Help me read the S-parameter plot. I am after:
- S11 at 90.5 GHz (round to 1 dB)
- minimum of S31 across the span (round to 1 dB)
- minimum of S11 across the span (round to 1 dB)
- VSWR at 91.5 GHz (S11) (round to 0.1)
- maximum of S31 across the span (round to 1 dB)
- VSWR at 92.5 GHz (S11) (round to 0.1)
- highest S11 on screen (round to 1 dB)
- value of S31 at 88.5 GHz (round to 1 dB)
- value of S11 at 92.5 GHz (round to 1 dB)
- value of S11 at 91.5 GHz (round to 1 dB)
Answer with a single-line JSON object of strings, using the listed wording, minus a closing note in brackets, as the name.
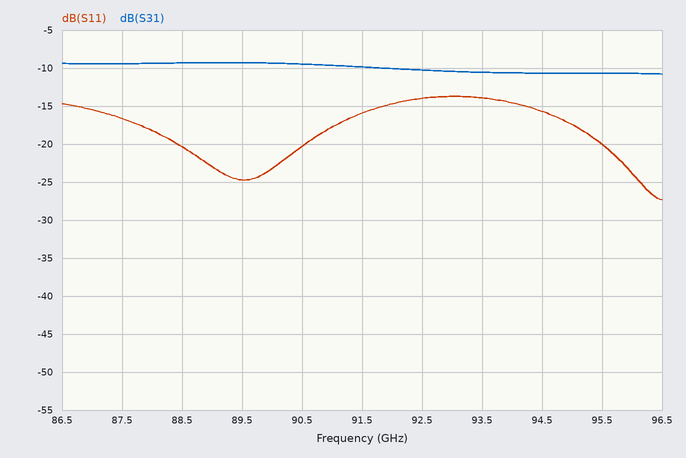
{"S11 at 90.5 GHz": "-20 dB", "minimum of S31 across the span": "-11 dB", "minimum of S11 across the span": "-27 dB", "VSWR at 91.5 GHz (S11)": "1.4", "maximum of S31 across the span": "-9 dB", "VSWR at 92.5 GHz (S11)": "1.5", "highest S11 on screen": "-14 dB", "value of S31 at 88.5 GHz": "-9 dB", "value of S11 at 92.5 GHz": "-14 dB", "value of S11 at 91.5 GHz": "-16 dB"}
